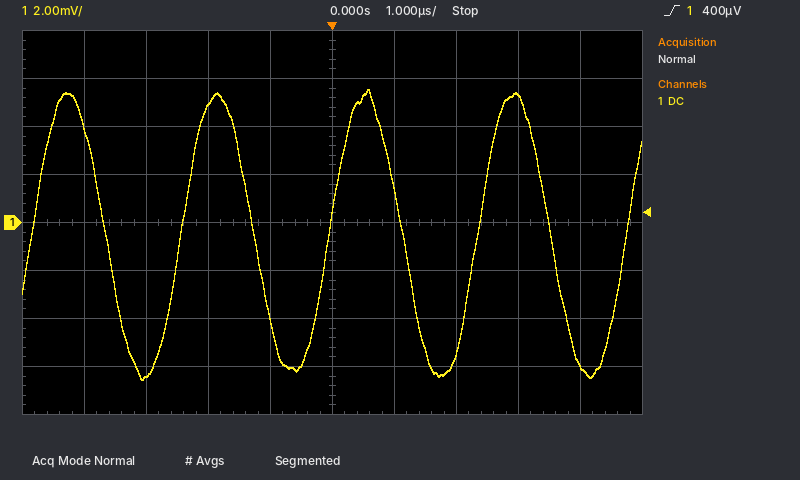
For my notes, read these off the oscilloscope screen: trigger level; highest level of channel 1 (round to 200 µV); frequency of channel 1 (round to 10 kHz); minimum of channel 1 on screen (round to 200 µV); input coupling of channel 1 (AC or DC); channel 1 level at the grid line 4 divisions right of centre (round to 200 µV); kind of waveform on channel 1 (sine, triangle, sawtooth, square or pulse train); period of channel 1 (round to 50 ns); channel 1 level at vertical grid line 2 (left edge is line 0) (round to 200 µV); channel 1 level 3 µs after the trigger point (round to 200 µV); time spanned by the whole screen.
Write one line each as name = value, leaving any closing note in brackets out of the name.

trigger level = 400 µV
highest level of channel 1 = 5.6 mV
frequency of channel 1 = 420 kHz
minimum of channel 1 on screen = -6.6 mV
input coupling of channel 1 = DC
channel 1 level at the grid line 4 divisions right of centre = -6.0 mV
kind of waveform on channel 1 = sine
period of channel 1 = 2.40 µs
channel 1 level at vertical grid line 2 (left edge is line 0) = -6.4 mV
channel 1 level 3 µs after the trigger point = 5.2 mV
time spanned by the whole screen = 10 µs
